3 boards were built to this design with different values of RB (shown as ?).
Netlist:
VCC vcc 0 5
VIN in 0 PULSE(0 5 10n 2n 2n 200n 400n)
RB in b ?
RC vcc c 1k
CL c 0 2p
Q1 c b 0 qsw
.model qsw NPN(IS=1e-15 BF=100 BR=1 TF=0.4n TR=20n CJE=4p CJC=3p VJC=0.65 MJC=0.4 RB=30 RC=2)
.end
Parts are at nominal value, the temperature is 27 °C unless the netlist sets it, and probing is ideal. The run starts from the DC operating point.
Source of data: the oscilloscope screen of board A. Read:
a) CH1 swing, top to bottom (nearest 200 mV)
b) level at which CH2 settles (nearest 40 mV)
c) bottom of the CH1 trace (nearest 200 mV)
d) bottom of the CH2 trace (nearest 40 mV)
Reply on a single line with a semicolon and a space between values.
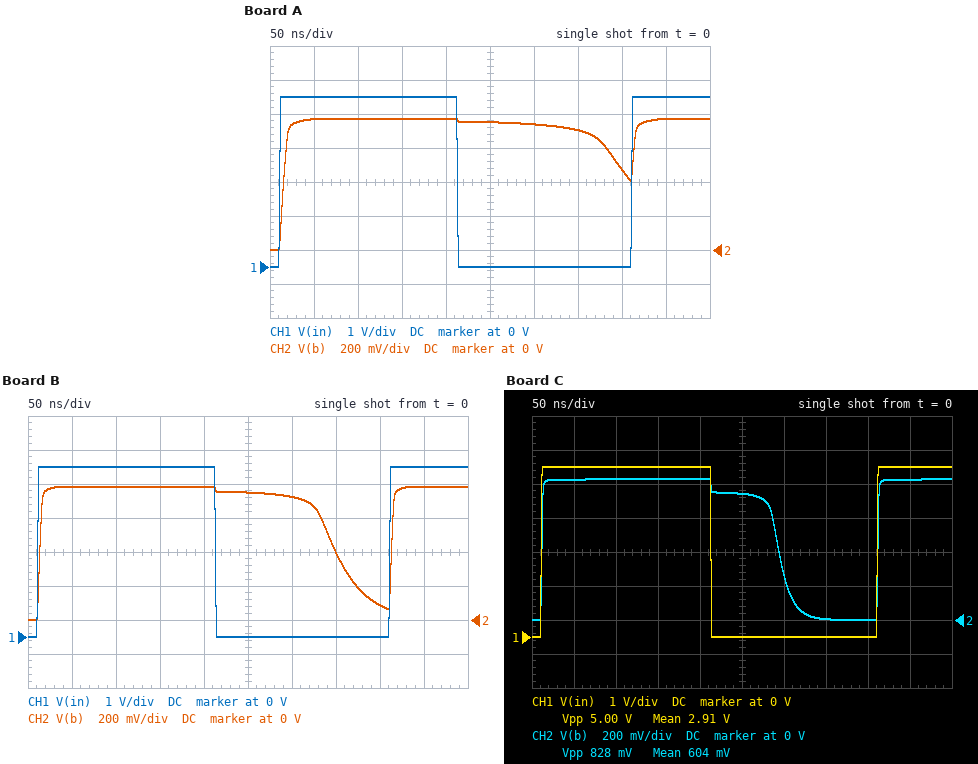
5.0 V; 760 mV; 0 V; 0 V
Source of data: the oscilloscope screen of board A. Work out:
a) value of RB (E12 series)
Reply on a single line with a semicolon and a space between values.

10 kΩ
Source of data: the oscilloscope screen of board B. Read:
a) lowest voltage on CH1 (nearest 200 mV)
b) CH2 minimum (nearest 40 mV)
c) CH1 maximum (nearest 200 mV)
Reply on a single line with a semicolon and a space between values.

0 V; 0 V; 5.0 V
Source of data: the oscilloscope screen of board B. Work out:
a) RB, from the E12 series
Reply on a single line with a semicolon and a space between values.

5.6 kΩ
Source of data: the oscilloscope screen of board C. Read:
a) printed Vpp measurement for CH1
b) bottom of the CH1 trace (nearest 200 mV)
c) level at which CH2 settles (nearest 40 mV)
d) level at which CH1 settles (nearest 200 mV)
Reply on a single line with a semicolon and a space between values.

5.00 V; 0 V; 840 mV; 5.0 V
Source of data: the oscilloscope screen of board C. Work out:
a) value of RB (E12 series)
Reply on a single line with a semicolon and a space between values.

2.2 kΩ
